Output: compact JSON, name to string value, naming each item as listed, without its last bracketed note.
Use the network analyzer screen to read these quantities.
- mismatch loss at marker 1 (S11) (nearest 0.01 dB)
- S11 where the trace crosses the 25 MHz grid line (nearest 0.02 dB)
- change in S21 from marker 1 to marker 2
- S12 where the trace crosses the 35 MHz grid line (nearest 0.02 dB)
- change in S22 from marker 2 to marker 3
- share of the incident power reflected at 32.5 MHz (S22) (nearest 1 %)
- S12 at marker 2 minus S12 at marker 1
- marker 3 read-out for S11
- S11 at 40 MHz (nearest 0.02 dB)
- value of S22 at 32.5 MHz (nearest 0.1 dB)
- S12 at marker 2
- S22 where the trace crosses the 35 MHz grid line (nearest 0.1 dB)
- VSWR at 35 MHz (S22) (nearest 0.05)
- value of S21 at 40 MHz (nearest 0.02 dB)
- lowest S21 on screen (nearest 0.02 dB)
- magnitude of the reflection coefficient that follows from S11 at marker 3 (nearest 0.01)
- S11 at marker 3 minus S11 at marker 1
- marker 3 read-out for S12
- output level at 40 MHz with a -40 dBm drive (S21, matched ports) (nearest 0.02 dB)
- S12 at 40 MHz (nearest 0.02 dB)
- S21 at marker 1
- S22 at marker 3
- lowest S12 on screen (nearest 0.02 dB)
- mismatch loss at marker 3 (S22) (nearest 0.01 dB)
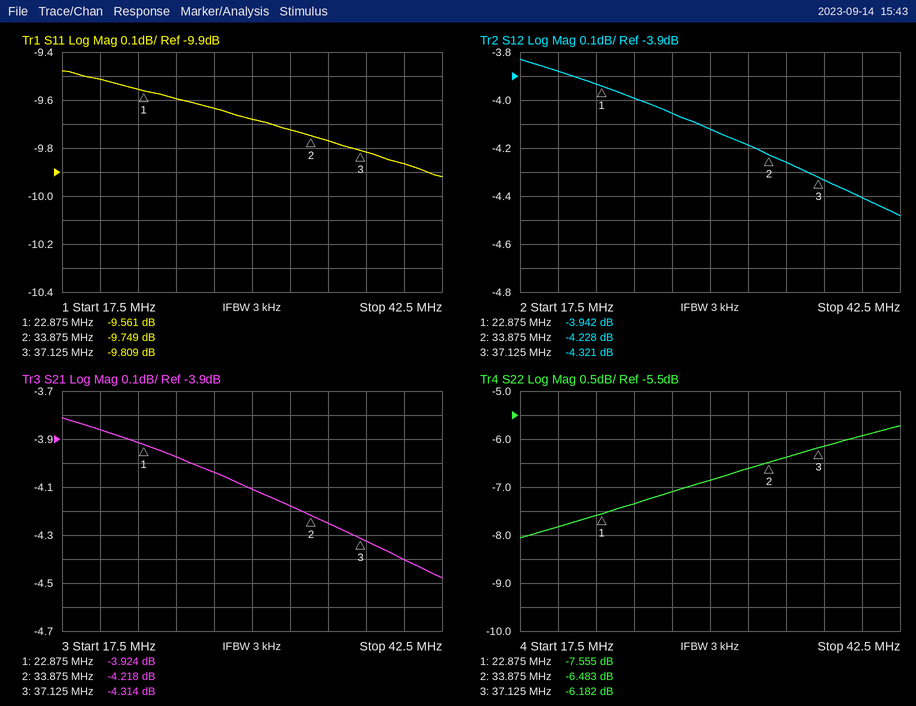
{"mismatch loss at marker 1 (S11)": "0.51 dB", "S11 where the trace crosses the 25 MHz grid line": "-9.60 dB", "change in S21 from marker 1 to marker 2": "-0.294 dB", "S12 where the trace crosses the 35 MHz grid line": "-4.26 dB", "change in S22 from marker 2 to marker 3": "0.301 dB", "share of the incident power reflected at 32.5 MHz (S22)": "22 %", "S12 at marker 2 minus S12 at marker 1": "-0.286 dB", "marker 3 read-out for S11": "-9.809 dB", "S11 at 40 MHz": "-9.86 dB", "value of S22 at 32.5 MHz": "-6.6 dB", "S12 at marker 2": "-4.228 dB", "S22 where the trace crosses the 35 MHz grid line": "-6.4 dB", "VSWR at 35 MHz (S22)": "2.85", "value of S21 at 40 MHz": "-4.40 dB", "lowest S21 on screen": "-4.48 dB", "magnitude of the reflection coefficient that follows from S11 at marker 3": "0.32", "S11 at marker 3 minus S11 at marker 1": "-0.248 dB", "marker 3 read-out for S12": "-4.321 dB", "output level at 40 MHz with a -40 dBm drive (S21, matched ports)": "-44.40 dBm", "S12 at 40 MHz": "-4.40 dB", "S21 at marker 1": "-3.924 dB", "S22 at marker 3": "-6.182 dB", "lowest S12 on screen": "-4.48 dB", "mismatch loss at marker 3 (S22)": "1.20 dB"}
